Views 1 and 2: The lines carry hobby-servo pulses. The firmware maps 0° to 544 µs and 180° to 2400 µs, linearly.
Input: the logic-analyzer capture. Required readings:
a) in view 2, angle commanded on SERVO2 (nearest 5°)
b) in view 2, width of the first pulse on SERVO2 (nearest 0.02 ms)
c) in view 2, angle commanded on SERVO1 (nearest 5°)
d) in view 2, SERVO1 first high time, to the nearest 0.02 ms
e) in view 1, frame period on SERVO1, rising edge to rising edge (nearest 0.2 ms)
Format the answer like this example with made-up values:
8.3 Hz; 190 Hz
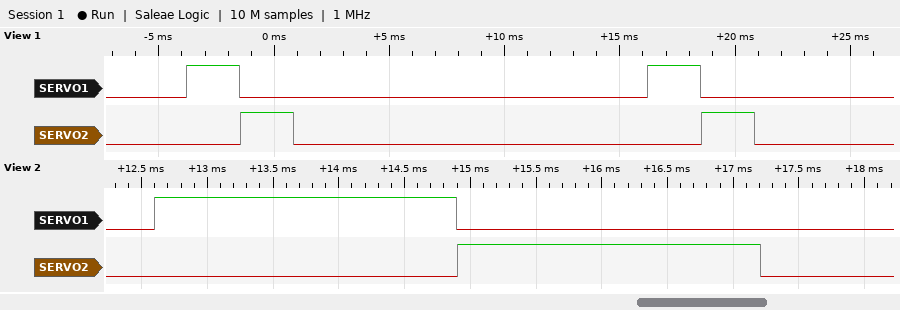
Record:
170°; 2.30 ms; 170°; 2.30 ms; 20.0 ms
